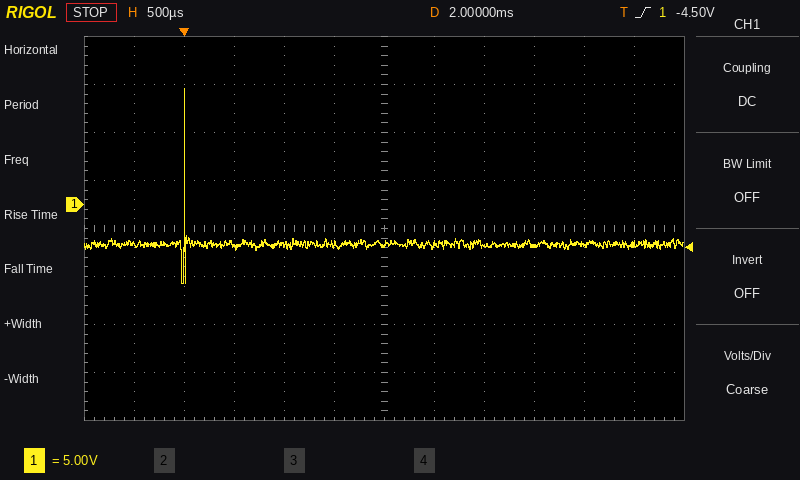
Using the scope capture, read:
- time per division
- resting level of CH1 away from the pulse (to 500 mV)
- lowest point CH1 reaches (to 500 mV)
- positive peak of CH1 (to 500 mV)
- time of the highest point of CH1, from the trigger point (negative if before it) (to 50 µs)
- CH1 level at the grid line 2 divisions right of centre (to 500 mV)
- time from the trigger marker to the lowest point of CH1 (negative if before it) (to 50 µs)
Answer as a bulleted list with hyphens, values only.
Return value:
- 500 µs
- -4.0 V
- -8.0 V
- 12.0 V
- 0 µs
- -4.5 V
- 0 µs
